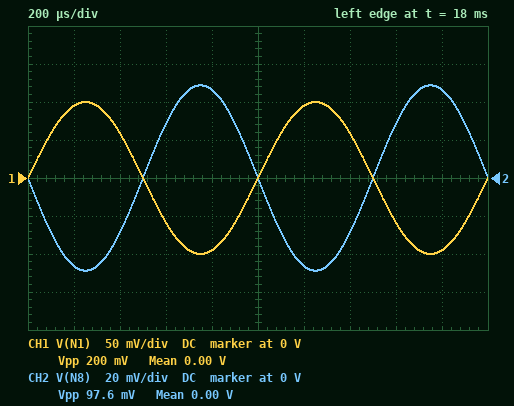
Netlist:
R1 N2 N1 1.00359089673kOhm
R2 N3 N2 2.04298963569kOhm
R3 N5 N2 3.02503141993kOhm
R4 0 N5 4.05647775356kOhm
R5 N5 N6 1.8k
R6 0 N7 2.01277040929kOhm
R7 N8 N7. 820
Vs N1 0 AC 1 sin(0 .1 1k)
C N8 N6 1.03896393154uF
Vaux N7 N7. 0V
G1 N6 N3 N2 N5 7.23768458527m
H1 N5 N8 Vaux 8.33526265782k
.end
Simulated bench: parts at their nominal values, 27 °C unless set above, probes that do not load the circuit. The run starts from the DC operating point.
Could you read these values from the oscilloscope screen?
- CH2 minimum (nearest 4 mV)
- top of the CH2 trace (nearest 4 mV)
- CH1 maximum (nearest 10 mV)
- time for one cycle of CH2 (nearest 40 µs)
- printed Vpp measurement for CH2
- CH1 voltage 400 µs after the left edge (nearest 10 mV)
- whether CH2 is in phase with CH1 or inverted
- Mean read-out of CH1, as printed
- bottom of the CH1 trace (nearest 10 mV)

-48 mV
48 mV
100 mV
1.00 ms
97.6 mV
60 mV
inverted
0.00 V
-100 mV
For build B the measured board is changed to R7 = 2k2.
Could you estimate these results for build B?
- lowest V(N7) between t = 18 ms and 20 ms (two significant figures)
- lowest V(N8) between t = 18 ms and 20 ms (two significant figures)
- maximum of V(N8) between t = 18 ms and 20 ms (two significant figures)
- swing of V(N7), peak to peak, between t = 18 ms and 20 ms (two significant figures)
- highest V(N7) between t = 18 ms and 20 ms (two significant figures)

-49 mV
-100 mV
100 mV
97 mV
49 mV
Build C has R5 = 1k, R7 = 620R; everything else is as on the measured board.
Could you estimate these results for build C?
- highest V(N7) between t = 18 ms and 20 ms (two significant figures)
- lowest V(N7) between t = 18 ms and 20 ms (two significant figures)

33 mV
-33 mV
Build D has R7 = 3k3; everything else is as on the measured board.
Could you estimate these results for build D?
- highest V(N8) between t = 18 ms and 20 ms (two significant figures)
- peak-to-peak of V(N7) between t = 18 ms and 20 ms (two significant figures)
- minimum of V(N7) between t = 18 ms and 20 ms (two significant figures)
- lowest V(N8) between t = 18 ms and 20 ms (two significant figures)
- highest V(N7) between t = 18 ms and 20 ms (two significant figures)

190 mV
140 mV
-72 mV
-190 mV
72 mV
